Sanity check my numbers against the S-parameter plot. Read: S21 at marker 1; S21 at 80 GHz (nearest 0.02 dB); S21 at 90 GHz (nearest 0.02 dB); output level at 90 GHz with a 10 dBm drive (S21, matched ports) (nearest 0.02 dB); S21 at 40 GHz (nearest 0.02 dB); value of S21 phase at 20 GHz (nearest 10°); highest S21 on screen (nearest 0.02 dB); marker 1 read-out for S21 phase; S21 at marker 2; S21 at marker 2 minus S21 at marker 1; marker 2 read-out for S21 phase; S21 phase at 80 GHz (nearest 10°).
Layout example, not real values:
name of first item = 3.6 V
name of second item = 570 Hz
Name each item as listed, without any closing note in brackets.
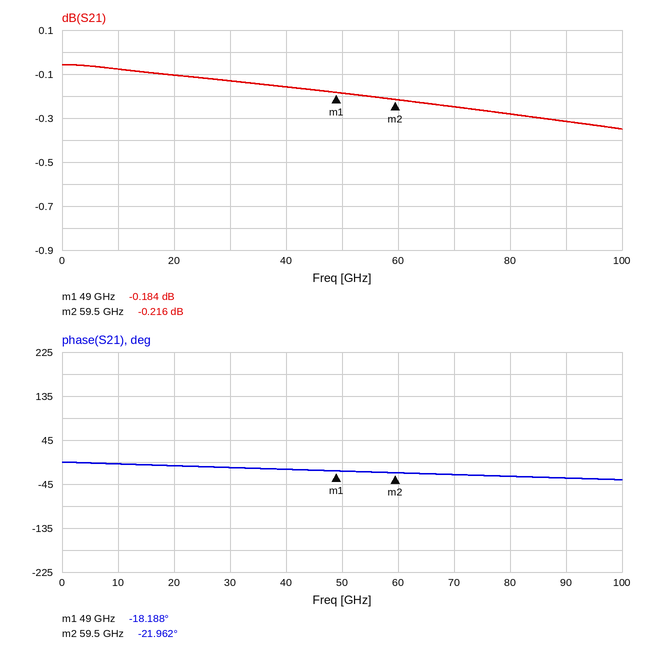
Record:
S21 at marker 1 = -0.184 dB
S21 at 80 GHz = -0.28 dB
S21 at 90 GHz = -0.32 dB
output level at 90 GHz with a 10 dBm drive (S21, matched ports) = 9.68 dBm
S21 at 40 GHz = -0.16 dB
value of S21 phase at 20 GHz = -10°
highest S21 on screen = -0.06 dB
marker 1 read-out for S21 phase = -18.188°
S21 at marker 2 = -0.216 dB
S21 at marker 2 minus S21 at marker 1 = -0.032 dB
marker 2 read-out for S21 phase = -21.962°
S21 phase at 80 GHz = -30°
